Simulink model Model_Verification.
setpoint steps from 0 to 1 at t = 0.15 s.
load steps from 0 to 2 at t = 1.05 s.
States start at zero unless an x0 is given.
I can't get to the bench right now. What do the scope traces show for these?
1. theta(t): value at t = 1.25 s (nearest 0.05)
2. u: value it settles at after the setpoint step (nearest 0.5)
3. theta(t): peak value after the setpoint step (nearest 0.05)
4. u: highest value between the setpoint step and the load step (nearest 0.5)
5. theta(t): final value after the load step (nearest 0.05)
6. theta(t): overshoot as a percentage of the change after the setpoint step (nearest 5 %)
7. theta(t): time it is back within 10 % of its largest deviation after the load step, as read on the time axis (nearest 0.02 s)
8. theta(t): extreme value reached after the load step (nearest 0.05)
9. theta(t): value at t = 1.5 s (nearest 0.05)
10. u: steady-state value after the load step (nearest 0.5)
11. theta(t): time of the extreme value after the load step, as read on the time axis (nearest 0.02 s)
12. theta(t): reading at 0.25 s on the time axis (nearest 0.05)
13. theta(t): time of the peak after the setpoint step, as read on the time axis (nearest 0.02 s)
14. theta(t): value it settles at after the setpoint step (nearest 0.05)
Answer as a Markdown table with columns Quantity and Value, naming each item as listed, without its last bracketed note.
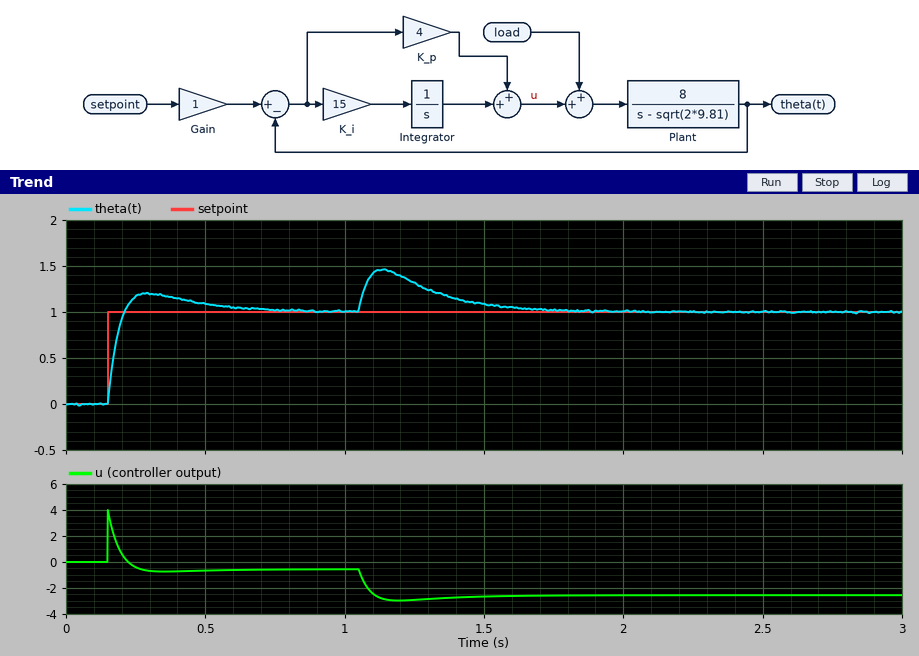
| Quantity | Value |
|---|---|
| theta(t): value at t = 1.25 s | 1.30 |
| u: value it settles at after the setpoint step | -0.5 |
| theta(t): peak value after the setpoint step | 1.20 |
| u: highest value between the setpoint step and the load step | 4.0 |
| theta(t): final value after the load step | 1.00 |
| theta(t): overshoot as a percentage of the change after the setpoint step | 20 % |
| theta(t): time it is back within 10 % of its largest deviation after the load step, as read on the time axis | 1.62 s |
| theta(t): extreme value reached after the load step | 1.45 |
| theta(t): value at t = 1.5 s | 1.10 |
| u: steady-state value after the load step | -2.5 |
| theta(t): time of the extreme value after the load step, as read on the time axis | 1.14 s |
| theta(t): reading at 0.25 s on the time axis | 1.15 |
| theta(t): time of the peak after the setpoint step, as read on the time axis | 0.30 s |
| theta(t): value it settles at after the setpoint step | 1.00 |
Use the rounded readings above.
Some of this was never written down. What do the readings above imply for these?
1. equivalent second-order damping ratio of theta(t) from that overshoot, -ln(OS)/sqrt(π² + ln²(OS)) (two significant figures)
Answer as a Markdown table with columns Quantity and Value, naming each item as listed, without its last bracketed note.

| Quantity | Value |
|---|---|
| equivalent second-order damping ratio of theta(t) from that overshoot, -ln(OS)/sqrt(π² + ln²(OS)) | 0.46 |
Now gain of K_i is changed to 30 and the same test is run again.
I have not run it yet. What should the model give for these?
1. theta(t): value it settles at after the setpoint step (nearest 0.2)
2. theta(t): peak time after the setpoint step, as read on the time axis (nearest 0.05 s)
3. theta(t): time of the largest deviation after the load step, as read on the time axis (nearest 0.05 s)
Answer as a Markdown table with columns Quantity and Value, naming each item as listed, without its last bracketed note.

| Quantity | Value |
|---|---|
| theta(t): value it settles at after the setpoint step | 1.0 |
| theta(t): peak time after the setpoint step, as read on the time axis | 0.25 s |
| theta(t): time of the largest deviation after the load step, as read on the time axis | 1.10 s |
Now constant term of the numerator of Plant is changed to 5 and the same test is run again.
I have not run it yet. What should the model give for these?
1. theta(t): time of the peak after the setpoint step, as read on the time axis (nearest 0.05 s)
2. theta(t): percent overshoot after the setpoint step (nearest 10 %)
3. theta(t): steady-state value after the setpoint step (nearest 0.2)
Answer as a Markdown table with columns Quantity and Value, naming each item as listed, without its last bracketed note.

| Quantity | Value |
|---|---|
| theta(t): time of the peak after the setpoint step, as read on the time axis | 0.35 s |
| theta(t): percent overshoot after the setpoint step | 30 % |
| theta(t): steady-state value after the setpoint step | 1.0 |
